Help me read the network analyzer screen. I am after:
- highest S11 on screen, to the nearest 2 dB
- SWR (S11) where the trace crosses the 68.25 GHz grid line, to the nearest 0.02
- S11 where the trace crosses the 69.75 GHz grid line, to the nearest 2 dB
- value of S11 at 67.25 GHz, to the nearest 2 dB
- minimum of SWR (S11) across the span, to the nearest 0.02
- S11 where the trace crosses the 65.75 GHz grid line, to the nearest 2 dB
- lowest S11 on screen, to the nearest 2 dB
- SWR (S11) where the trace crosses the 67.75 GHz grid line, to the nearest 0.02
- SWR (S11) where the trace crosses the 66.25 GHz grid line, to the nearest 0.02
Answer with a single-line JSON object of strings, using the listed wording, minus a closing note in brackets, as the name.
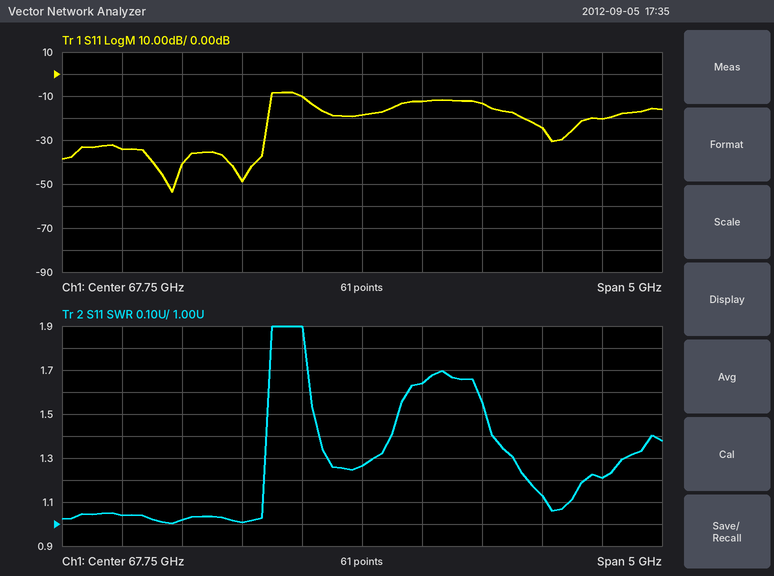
{"highest S11 on screen, to the nearest 2 dB": "-8 dB", "SWR (S11) where the trace crosses the 68.25 GHz grid line, to the nearest 0.02": "1.64", "S11 where the trace crosses the 69.75 GHz grid line, to the nearest 2 dB": "-20 dB", "value of S11 at 67.25 GHz, to the nearest 2 dB": "-10 dB", "minimum of SWR (S11) across the span, to the nearest 0.02": "1.00", "S11 where the trace crosses the 65.75 GHz grid line, to the nearest 2 dB": "-34 dB", "lowest S11 on screen, to the nearest 2 dB": "-54 dB", "SWR (S11) where the trace crosses the 67.75 GHz grid line, to the nearest 0.02": "1.26", "SWR (S11) where the trace crosses the 66.25 GHz grid line, to the nearest 0.02": "1.02"}
